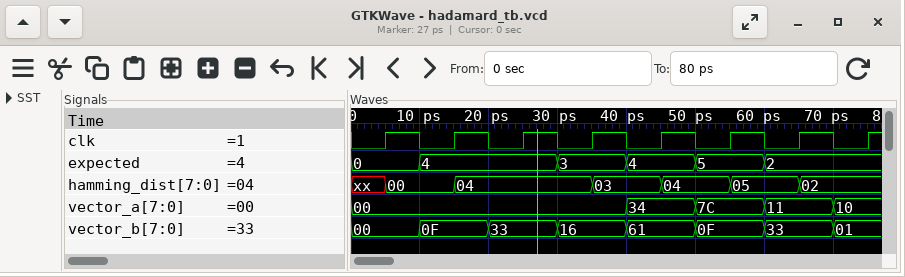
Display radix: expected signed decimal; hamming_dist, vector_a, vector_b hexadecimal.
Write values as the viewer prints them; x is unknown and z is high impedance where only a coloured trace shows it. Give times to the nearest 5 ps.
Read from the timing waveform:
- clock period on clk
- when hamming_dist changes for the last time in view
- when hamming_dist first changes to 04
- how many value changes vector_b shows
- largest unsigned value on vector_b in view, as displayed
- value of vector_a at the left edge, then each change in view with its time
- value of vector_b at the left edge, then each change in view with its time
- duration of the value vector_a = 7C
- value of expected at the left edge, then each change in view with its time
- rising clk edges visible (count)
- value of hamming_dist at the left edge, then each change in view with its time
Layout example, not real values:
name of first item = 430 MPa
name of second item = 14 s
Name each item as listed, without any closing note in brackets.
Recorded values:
clock period on clk = 10 ps
when hamming_dist changes for the last time in view = 65 ps
when hamming_dist first changes to 04 = 15 ps
how many value changes vector_b shows = 7
largest unsigned value on vector_b in view, as displayed = 61
value of vector_a at the left edge, then each change in view with its time = 00, 34 at 40 ps, 7C at 50 ps, 11 at 60 ps, 10 at 70 ps
value of vector_b at the left edge, then each change in view with its time = 00, 0F at 10 ps, 33 at 20 ps, 16 at 30 ps, 61 at 40 ps, 0F at 50 ps, 33 at 60 ps, 01 at 70 ps
duration of the value vector_a = 7C = 10 ps
value of expected at the left edge, then each change in view with its time = 0, 4 at 10 ps, 3 at 30 ps, 4 at 40 ps, 5 at 50 ps, 2 at 60 ps
rising clk edges visible = 8
value of hamming_dist at the left edge, then each change in view with its time = xx, 00 at 5 ps, 04 at 15 ps, 03 at 35 ps, 04 at 45 ps, 05 at 55 ps, 02 at 65 ps
